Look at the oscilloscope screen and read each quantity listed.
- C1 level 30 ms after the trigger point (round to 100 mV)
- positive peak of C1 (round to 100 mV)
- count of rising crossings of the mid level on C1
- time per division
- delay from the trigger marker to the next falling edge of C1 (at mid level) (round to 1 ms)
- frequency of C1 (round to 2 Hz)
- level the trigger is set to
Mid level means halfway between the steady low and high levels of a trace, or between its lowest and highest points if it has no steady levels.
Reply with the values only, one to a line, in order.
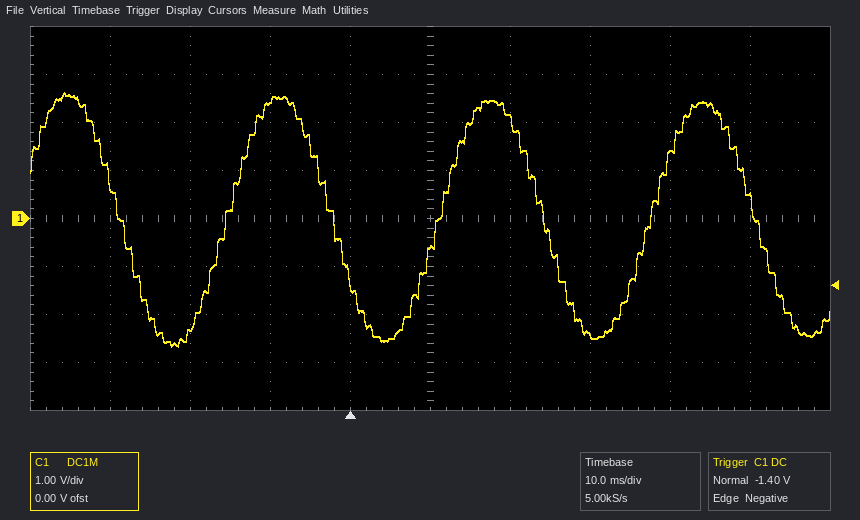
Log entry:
-2.4 V
2.6 V
3
10 ms
24 ms
38 Hz
-1.40 V
